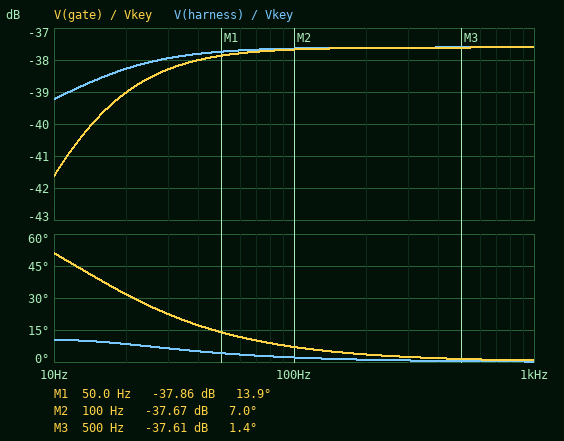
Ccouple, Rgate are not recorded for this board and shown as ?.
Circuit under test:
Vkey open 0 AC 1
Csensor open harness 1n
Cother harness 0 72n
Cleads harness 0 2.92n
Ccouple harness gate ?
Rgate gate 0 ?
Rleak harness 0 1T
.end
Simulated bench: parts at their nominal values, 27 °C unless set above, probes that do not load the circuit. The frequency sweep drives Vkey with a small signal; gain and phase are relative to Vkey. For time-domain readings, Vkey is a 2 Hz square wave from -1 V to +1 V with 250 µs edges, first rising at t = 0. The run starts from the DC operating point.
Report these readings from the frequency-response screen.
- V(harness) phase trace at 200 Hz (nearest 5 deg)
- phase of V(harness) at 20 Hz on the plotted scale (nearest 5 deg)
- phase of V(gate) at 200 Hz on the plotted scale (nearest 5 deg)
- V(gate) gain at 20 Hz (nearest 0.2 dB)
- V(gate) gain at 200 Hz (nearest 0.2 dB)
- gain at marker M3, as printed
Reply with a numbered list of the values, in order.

1. 0 deg
2. 10 deg
3. 5 deg
4. -39.0 dB
5. -37.6 dB
6. -37.61 dB
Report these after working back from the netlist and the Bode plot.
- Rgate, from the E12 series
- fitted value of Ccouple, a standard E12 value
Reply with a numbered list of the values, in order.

1. 560 kΩ
2. 33 nF
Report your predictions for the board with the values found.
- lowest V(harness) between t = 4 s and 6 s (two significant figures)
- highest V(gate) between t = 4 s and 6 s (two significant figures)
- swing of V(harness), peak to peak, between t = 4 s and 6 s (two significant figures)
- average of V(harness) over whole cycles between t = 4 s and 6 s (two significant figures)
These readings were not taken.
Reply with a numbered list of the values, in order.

1. -7.9 mV
2. 26 mV
3. 34 mV
4. 9.2 mV
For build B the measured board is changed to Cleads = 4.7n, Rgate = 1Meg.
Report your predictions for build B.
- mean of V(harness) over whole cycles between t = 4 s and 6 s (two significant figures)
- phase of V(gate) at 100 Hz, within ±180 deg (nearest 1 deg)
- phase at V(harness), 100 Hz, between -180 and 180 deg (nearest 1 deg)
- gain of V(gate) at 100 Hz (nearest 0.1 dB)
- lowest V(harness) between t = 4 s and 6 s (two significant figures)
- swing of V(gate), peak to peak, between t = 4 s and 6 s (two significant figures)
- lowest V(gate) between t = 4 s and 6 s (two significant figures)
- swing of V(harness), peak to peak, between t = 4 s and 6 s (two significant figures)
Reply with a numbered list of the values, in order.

1. 9.0 mV
2. 4 deg
3. 1 deg
4. -37.8 dB
5. -7.6 mV
6. 51 mV
7. -26 mV
8. 33 mV
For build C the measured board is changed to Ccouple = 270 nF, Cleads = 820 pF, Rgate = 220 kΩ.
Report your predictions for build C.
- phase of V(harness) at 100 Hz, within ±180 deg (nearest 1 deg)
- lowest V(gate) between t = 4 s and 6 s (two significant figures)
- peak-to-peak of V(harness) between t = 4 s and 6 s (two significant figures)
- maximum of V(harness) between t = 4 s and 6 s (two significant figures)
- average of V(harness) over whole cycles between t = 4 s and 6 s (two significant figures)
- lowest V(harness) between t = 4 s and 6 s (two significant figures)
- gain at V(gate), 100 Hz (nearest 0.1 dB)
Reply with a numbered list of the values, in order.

1. 6 deg
2. -27 mV
3. 48 mV
4. 27 mV
5. 2.9 mV
6. -21 mV
7. -37.4 dB
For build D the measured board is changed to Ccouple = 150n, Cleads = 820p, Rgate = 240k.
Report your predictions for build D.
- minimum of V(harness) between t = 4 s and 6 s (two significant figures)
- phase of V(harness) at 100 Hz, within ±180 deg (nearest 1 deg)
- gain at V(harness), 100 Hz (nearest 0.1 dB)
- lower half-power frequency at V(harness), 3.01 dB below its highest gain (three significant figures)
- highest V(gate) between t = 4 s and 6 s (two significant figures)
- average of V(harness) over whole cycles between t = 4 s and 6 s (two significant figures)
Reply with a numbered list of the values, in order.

1. -18 mV
2. 5 deg
3. -37.4 dB
4. 11.9 Hz
5. 27 mV
6. 4.5 mV
